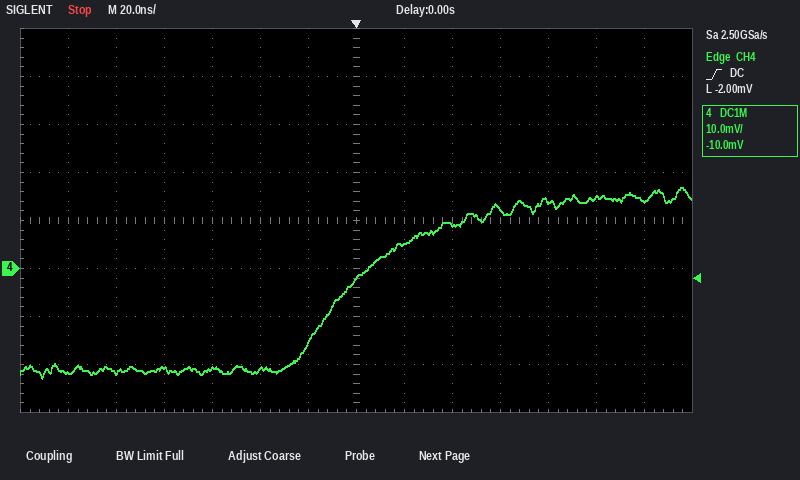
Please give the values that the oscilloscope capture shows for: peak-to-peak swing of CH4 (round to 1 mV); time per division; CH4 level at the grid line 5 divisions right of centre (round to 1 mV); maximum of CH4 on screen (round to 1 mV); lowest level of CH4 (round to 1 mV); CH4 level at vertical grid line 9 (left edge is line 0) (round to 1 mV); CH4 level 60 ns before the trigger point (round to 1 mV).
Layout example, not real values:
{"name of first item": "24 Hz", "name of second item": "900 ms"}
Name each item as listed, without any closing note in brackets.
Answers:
{"peak-to-peak swing of CH4": "40 mV", "time per division": "20 ns", "CH4 level at the grid line 5 divisions right of centre": "15 mV", "maximum of CH4 on screen": "17 mV", "lowest level of CH4": "-23 mV", "CH4 level at vertical grid line 9 (left edge is line 0)": "9 mV", "CH4 level 60 ns before the trigger point": "-21 mV"}
